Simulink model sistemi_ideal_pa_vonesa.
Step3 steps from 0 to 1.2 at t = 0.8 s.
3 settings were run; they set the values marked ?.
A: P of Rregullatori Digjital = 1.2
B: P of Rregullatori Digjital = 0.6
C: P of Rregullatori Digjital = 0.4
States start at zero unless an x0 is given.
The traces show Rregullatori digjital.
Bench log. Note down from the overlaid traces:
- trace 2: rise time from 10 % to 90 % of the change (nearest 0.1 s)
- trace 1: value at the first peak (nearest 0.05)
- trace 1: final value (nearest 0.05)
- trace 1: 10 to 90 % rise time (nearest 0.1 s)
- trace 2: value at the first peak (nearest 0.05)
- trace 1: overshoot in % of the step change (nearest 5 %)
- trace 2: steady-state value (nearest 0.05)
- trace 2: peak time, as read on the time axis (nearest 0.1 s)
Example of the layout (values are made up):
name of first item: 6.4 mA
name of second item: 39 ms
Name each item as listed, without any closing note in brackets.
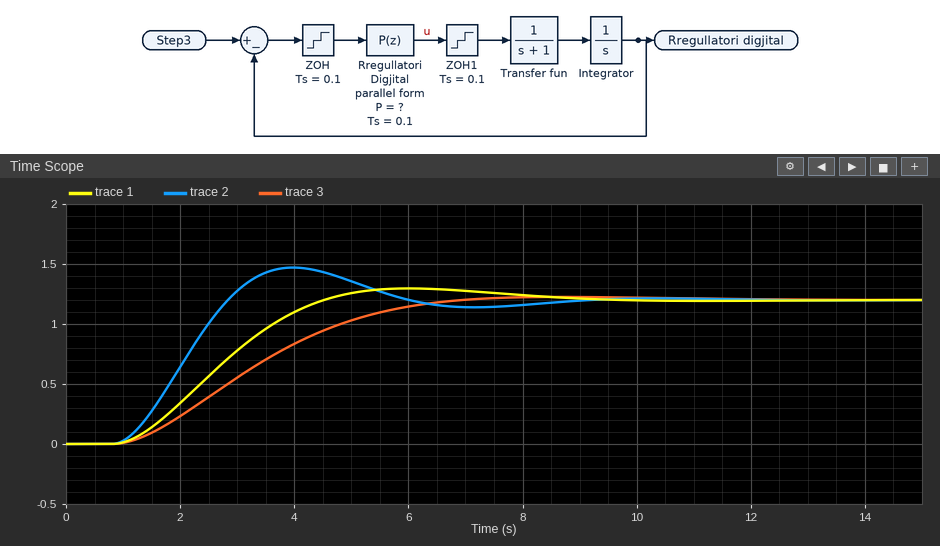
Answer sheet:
trace 2: rise time from 10 % to 90 % of the change: 1.4 s
trace 1: value at the first peak: 1.30
trace 1: final value: 1.20
trace 1: 10 to 90 % rise time: 2.5 s
trace 2: value at the first peak: 1.45
trace 1: overshoot in % of the step change: 10 %
trace 2: steady-state value: 1.20
trace 2: peak time, as read on the time axis: 4.0 s
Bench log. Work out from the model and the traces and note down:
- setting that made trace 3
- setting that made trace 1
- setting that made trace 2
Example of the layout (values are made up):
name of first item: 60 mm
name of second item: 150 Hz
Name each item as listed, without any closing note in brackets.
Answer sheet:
setting that made trace 3: C
setting that made trace 1: B
setting that made trace 2: A
